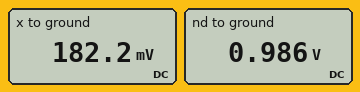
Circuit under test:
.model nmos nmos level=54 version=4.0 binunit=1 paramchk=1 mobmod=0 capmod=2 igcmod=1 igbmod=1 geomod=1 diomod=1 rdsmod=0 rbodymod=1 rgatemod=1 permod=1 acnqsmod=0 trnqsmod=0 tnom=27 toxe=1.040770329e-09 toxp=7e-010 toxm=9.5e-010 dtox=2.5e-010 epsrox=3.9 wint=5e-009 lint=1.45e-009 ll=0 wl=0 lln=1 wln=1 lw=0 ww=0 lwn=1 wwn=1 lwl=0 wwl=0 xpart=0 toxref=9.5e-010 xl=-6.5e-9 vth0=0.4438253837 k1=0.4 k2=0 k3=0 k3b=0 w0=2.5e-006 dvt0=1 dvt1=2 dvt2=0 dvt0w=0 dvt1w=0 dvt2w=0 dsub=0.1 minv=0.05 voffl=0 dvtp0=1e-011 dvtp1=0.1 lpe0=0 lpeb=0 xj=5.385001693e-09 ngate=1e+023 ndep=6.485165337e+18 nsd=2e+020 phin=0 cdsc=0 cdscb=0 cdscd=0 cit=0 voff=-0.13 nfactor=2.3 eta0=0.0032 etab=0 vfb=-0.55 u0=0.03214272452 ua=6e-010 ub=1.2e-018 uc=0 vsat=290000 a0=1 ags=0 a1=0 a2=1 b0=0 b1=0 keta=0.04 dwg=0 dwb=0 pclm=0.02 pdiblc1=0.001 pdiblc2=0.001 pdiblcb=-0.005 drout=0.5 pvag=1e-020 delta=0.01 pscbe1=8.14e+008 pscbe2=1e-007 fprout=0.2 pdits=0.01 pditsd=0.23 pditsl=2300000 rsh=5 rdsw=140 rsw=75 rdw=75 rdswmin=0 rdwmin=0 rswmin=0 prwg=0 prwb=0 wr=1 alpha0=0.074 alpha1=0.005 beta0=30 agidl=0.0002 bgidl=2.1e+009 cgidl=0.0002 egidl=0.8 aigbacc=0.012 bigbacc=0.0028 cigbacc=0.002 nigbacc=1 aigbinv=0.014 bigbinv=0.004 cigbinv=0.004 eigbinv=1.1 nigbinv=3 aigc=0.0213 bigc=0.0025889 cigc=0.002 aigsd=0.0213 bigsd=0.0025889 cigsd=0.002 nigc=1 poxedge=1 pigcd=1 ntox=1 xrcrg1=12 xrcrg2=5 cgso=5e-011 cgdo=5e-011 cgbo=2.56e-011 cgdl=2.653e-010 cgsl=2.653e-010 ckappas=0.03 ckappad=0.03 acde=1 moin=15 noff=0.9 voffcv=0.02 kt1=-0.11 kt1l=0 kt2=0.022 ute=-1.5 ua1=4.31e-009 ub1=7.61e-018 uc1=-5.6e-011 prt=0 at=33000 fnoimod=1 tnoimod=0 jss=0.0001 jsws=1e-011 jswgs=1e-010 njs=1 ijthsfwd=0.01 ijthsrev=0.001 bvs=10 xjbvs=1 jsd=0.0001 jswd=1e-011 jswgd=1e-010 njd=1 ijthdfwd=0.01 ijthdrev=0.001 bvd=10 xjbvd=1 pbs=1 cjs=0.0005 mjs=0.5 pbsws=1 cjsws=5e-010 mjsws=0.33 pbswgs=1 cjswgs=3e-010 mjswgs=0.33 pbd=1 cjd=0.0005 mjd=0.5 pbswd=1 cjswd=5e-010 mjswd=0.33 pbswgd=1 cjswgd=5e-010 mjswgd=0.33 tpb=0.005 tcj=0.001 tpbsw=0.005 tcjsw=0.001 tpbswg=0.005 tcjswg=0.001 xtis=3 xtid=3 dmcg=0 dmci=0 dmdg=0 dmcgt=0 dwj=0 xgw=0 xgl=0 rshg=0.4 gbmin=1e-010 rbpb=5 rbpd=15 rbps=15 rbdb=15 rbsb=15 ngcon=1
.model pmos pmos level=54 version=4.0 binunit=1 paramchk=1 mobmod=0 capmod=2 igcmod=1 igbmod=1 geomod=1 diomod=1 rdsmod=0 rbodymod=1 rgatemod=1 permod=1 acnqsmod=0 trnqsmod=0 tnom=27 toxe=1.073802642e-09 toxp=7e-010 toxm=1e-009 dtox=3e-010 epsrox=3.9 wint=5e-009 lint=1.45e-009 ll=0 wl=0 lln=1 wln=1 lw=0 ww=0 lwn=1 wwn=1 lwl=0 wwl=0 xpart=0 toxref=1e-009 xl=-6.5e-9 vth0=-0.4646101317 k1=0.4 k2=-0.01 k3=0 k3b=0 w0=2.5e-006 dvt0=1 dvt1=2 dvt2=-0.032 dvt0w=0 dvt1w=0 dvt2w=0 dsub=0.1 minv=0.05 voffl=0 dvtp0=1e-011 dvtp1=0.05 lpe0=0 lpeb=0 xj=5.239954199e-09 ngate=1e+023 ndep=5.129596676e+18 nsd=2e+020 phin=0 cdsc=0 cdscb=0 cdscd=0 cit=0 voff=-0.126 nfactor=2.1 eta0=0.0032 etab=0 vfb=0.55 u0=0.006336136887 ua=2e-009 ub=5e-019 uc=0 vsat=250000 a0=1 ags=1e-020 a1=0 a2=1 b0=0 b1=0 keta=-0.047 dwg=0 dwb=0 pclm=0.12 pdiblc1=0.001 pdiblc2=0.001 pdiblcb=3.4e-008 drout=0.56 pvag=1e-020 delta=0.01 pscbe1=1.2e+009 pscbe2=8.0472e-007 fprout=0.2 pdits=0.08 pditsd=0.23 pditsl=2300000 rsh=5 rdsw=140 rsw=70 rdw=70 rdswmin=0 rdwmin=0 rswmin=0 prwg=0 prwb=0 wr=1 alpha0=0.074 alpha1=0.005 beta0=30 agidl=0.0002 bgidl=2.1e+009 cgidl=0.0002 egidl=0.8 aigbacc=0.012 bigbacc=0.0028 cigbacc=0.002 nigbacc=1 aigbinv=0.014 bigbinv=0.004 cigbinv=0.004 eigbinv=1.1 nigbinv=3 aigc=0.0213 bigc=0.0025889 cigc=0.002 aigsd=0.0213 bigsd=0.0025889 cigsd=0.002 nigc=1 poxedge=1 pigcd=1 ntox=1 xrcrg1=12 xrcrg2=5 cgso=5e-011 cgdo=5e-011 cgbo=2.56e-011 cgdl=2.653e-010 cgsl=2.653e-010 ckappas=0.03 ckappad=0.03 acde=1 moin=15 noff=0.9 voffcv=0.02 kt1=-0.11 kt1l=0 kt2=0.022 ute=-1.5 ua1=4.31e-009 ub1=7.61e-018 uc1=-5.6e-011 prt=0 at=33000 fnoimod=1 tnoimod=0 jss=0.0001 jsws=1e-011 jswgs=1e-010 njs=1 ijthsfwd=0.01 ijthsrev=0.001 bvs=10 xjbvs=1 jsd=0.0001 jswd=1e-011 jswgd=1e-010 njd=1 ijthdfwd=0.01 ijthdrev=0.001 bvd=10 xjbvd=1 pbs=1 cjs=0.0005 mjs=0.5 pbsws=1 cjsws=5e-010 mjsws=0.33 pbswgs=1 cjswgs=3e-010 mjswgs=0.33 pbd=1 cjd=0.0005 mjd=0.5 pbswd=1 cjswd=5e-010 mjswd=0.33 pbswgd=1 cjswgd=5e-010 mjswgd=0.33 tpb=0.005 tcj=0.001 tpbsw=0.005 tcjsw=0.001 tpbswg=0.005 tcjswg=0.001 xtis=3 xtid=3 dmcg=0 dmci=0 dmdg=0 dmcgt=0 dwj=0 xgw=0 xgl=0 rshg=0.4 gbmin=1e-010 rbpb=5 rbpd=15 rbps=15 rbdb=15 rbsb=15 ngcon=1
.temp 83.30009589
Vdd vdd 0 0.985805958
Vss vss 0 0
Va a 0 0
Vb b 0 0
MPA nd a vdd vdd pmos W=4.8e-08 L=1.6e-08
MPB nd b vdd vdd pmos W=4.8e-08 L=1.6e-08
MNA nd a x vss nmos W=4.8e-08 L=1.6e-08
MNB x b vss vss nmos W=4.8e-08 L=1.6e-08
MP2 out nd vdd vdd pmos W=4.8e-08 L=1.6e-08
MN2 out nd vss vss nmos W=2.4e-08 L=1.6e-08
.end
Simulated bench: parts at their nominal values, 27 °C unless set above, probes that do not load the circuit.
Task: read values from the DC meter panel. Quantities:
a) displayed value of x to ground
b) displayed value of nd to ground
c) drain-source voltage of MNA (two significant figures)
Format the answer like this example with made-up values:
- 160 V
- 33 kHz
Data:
- 182.2 mV
- 0.986 V
- 800 mV
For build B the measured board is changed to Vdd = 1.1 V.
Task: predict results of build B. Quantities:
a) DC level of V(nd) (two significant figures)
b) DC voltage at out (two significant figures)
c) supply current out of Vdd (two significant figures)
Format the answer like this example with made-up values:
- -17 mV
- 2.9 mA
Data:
- 1.1 V
- 13 mV
- 1.2 µA
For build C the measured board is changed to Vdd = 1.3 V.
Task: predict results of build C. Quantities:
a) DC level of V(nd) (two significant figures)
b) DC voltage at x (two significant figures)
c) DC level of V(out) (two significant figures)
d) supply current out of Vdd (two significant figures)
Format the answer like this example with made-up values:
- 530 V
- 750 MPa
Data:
- 1.3 V
- 250 mV
- 61 mV
- 5.6 µA
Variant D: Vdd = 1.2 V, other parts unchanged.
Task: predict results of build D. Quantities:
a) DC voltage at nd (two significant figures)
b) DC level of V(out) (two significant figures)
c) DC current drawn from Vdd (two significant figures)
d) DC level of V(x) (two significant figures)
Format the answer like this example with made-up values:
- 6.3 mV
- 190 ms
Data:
- 1.2 V
- 30 mV
- 2.8 µA
- 230 mV
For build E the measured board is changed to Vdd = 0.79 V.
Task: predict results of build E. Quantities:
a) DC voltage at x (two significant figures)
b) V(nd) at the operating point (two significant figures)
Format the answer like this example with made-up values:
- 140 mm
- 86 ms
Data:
- 140 mV
- 790 mV
